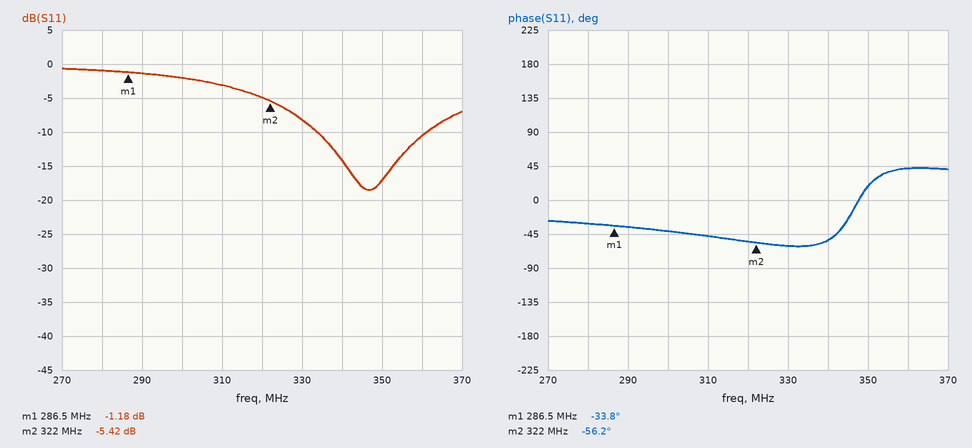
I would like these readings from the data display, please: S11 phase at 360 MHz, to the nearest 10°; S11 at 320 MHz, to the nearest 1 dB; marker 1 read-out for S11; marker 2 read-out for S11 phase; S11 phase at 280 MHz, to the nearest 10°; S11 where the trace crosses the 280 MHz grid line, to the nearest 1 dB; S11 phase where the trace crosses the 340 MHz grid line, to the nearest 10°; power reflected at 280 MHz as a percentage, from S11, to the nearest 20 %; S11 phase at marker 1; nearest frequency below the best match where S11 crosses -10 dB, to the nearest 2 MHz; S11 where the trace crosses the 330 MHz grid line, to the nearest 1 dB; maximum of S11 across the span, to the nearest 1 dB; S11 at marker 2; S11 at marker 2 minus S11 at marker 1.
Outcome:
40°
-5 dB
-1.18 dB
-56.2°
-30°
-1 dB
-50°
80 %
-33.8°
334 MHz
-8 dB
-1 dB
-5.42 dB
-4.24 dB
